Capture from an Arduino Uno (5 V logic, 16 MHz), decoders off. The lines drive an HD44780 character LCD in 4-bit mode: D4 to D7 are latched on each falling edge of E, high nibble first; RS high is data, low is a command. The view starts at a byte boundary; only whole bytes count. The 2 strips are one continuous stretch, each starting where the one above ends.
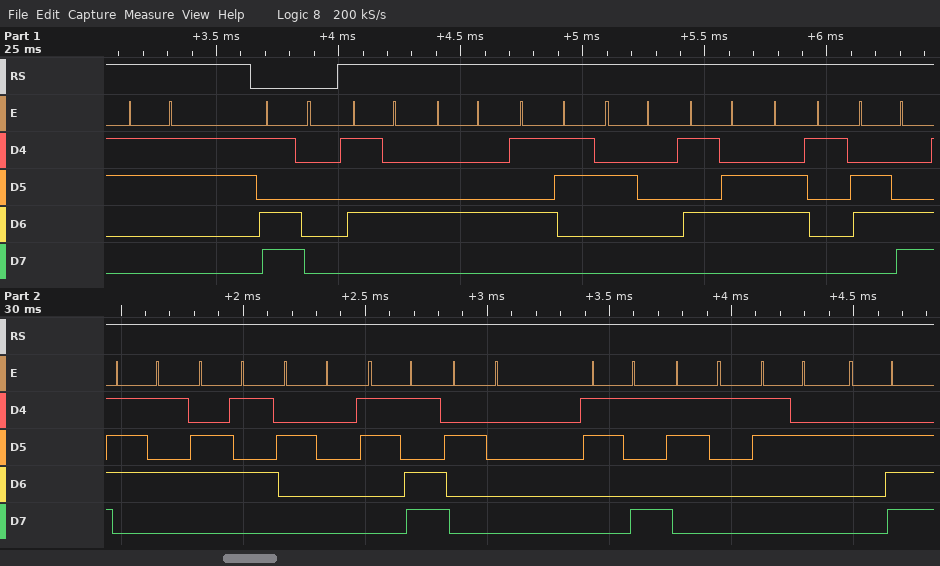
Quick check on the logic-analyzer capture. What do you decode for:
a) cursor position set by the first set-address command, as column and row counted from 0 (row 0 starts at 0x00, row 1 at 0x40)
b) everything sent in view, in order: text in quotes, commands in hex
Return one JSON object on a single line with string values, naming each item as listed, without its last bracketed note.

{"cursor position set by the first set-address command, as column and row counted from 0": "column 16, row 1", "everything sent in view, in order: text in quotes, commands in hex": "\"3\" 0xD0 \"TDS Value = 912.\""}
